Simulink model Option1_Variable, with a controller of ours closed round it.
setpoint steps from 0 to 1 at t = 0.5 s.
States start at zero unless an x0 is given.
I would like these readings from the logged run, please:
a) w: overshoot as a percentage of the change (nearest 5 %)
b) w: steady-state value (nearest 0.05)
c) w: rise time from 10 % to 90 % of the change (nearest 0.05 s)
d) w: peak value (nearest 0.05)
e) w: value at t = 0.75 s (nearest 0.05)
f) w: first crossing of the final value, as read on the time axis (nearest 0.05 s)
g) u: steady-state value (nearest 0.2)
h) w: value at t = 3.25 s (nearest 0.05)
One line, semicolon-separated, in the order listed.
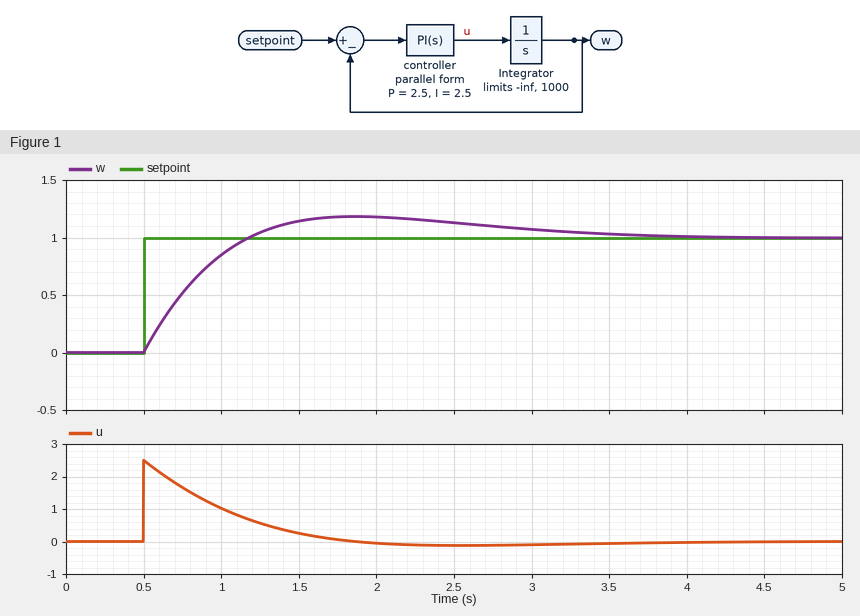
20 %; 1.00; 0.50 s; 1.20; 0.50; 1.20 s; 0.0; 1.05
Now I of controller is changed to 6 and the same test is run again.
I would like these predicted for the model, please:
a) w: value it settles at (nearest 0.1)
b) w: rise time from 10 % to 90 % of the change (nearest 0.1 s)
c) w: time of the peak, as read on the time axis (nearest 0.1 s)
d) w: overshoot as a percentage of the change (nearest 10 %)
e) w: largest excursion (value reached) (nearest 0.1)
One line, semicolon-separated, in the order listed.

1.0; 0.4 s; 1.5 s; 30 %; 1.3
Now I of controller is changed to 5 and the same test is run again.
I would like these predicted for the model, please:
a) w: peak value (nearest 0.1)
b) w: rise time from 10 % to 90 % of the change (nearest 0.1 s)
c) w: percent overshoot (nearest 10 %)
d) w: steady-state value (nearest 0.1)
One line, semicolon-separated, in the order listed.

1.3; 0.4 s; 30 %; 1.0
